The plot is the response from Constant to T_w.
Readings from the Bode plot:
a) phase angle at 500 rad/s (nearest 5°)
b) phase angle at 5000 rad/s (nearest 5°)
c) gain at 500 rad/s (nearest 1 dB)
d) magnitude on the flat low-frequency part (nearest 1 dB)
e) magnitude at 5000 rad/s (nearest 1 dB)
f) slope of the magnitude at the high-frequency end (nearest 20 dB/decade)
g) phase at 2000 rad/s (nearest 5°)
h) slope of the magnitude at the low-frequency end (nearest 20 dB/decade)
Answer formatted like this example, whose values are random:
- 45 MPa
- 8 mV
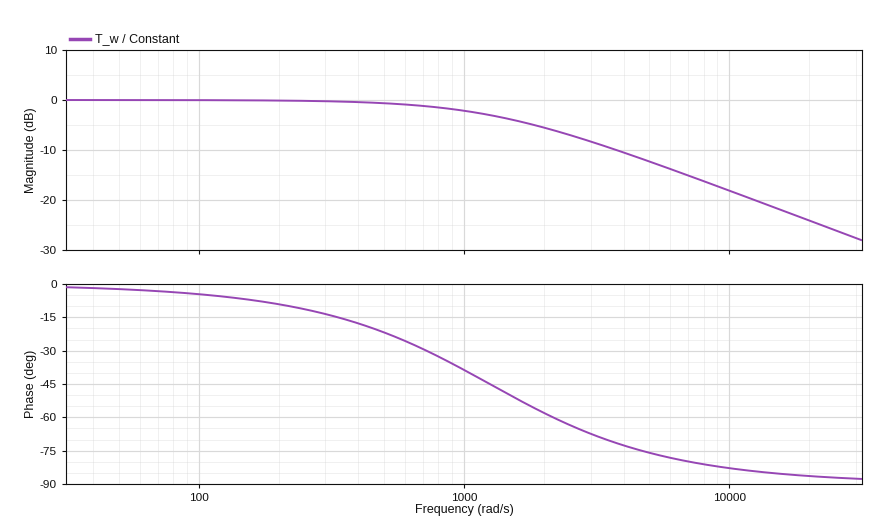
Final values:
- -20°
- -75°
- -1 dB
- 0 dB
- -12 dB
- -20 dB/decade
- -60°
- 0 dB/decade
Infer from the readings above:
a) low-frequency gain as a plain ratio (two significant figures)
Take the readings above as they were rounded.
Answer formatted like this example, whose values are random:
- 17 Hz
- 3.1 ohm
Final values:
- 1.0
